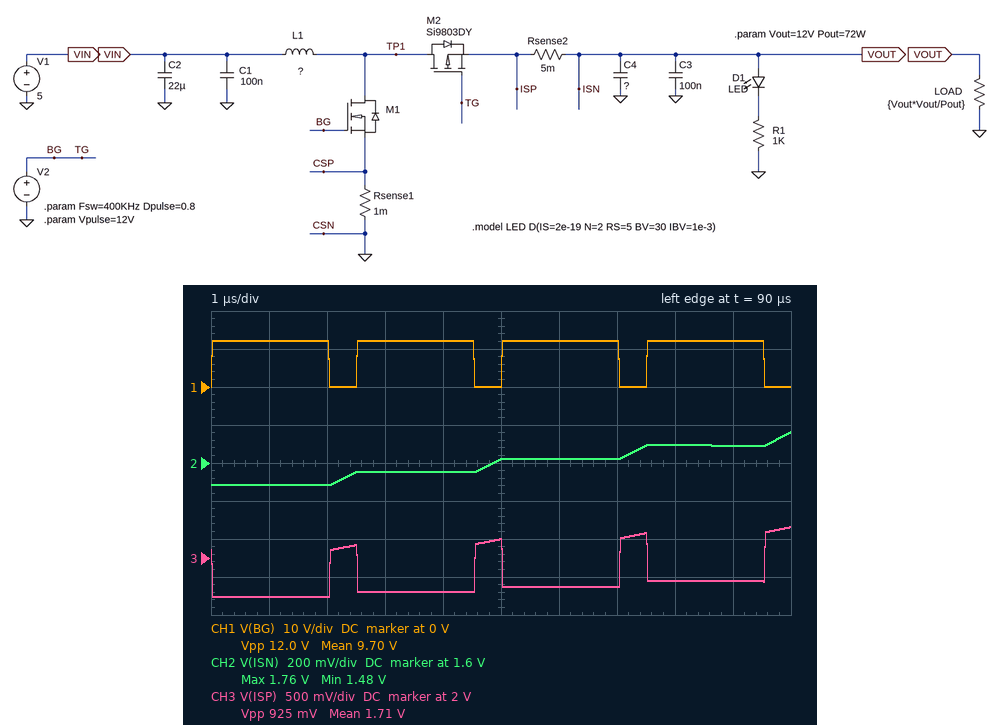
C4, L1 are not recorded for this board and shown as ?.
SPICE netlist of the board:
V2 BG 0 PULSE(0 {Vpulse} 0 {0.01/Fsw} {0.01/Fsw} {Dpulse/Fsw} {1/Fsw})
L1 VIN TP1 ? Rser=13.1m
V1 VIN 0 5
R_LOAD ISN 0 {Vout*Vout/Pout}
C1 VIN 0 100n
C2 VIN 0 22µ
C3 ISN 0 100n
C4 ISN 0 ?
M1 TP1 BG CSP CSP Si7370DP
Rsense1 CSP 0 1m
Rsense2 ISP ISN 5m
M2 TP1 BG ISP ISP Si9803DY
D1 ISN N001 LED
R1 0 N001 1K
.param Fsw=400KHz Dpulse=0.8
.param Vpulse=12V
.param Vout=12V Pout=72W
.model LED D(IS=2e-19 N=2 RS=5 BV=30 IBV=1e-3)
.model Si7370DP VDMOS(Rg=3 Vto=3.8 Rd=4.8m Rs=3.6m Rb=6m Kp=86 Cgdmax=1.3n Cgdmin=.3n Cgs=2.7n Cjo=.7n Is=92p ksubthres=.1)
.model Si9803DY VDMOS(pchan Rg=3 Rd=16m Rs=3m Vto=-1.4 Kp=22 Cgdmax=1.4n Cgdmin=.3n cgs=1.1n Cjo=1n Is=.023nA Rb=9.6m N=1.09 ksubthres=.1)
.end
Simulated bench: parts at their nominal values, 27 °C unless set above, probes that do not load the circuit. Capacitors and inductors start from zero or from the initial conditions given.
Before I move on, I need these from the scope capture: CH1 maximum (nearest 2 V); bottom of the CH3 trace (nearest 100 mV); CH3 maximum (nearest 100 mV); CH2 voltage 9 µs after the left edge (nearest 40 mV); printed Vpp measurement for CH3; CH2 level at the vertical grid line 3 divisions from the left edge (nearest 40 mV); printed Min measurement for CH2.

12 V
1.5 V
2.4 V
1.68 V
925 mV
1.56 V
1.48 V
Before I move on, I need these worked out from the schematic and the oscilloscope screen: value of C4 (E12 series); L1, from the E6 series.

820 µF
2.2 µH
